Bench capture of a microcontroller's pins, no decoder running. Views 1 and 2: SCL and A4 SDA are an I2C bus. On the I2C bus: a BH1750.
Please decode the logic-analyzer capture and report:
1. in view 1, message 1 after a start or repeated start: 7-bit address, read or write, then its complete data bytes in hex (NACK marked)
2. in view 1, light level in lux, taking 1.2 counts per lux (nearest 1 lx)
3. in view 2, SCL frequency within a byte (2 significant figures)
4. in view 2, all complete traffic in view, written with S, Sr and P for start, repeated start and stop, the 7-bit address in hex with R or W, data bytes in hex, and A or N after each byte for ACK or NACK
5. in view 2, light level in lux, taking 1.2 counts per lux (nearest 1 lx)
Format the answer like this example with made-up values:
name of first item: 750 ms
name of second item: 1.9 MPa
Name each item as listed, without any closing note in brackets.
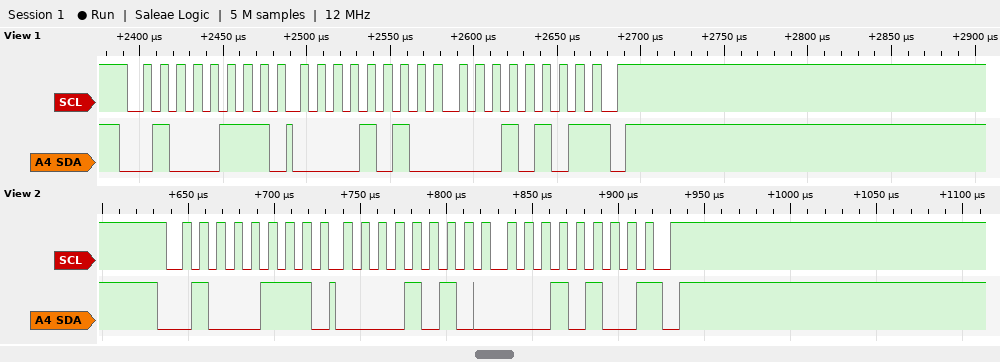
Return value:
in view 1, message 1 after a start or repeated start: 7-bit address, read or write, then its complete data bytes in hex: 0x23 read: 0A 15 NACK
in view 1, light level in lux, taking 1.2 counts per lux: 2151 lx
in view 2, SCL frequency within a byte: 100 kHz
in view 2, all complete traffic in view, written with S, Sr and P for start, repeated start and stop, the 7-bit address in hex with R or W, data bytes in hex, and A or N after each byte for ACK or NACK: S 23R A 0A A 14 N P
in view 2, light level in lux, taking 1.2 counts per lux: 2150 lx
